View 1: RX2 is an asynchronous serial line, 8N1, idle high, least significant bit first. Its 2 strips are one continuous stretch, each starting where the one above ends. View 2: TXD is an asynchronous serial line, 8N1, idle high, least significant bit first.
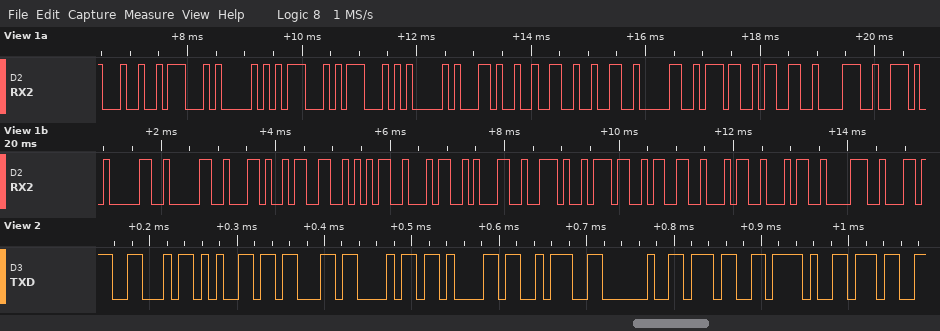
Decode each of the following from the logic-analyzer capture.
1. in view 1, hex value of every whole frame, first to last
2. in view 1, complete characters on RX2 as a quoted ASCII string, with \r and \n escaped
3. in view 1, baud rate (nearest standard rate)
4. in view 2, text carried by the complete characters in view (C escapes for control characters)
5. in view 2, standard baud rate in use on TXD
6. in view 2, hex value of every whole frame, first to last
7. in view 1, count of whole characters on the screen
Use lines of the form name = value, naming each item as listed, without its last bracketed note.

in view 1, hex value of every whole frame, first to last = 24 47 50 47 47 41 2C 32 32 30 37 33 38 2E 30 30 2C 33 35 34 31 2E 37 33 34 34 38
in view 1, complete characters on RX2 as a quoted ASCII string, with \r and \n escaped = "$GPGGA,220738.00,3541.73448"
in view 1, baud rate = 9600 baud
in view 2, text carried by the complete characters in view = "Fecha: 7/7"
in view 2, standard baud rate in use on TXD = 115200 baud
in view 2, hex value of every whole frame, first to last = 46 65 63 68 61 3A 20 37 2F 37
in view 1, count of whole characters on the screen = 27
